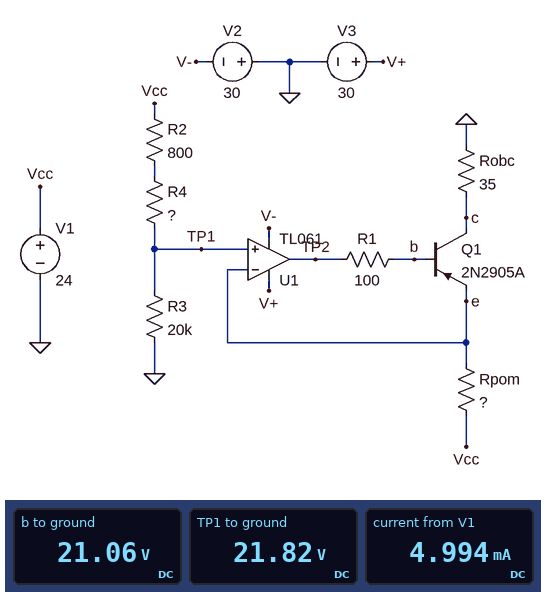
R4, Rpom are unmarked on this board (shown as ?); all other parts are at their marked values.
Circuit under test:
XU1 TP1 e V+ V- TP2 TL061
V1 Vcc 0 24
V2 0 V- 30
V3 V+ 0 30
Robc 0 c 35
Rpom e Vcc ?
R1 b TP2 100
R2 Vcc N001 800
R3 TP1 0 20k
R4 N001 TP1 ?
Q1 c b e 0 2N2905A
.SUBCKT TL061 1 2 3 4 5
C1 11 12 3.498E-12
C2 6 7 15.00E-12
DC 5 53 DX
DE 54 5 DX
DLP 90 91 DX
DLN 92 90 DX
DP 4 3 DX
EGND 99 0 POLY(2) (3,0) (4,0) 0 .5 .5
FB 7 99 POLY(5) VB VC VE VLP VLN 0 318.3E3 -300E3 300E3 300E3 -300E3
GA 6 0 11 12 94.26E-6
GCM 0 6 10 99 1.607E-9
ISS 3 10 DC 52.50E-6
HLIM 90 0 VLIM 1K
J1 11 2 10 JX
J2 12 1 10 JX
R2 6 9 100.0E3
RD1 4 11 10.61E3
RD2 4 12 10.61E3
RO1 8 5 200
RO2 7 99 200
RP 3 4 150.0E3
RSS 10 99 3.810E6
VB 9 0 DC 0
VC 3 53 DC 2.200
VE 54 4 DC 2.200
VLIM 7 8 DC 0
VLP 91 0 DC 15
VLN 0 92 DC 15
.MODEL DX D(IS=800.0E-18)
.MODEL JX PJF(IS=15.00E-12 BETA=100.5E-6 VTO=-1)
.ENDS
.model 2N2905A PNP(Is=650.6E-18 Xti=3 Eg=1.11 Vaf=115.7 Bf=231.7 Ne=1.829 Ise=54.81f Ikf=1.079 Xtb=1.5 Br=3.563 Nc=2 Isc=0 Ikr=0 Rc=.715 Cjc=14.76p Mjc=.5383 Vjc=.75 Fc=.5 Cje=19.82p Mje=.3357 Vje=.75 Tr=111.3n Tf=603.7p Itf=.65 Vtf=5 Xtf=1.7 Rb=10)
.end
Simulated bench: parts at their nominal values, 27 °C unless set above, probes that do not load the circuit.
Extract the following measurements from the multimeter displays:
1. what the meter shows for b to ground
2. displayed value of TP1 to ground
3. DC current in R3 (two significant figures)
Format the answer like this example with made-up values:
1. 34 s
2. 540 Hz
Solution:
1. 21.06 V
2. 21.82 V
3. 1.1 mA
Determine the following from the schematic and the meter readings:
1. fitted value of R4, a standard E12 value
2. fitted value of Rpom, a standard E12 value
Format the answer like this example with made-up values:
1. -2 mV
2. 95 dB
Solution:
1. 1.2 kΩ
2. 560 Ω
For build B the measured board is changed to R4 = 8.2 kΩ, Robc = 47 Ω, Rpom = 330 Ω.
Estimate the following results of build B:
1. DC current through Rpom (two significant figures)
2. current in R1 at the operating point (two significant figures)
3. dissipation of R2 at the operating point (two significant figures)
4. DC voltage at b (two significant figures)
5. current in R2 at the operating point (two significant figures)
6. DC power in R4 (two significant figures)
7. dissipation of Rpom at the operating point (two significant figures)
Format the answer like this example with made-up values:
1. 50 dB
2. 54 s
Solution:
1. 23 mA
2. 89 µA
3. 550 µW
4. 16 V
5. 830 µA
6. 5.6 mW
7. 170 mW
